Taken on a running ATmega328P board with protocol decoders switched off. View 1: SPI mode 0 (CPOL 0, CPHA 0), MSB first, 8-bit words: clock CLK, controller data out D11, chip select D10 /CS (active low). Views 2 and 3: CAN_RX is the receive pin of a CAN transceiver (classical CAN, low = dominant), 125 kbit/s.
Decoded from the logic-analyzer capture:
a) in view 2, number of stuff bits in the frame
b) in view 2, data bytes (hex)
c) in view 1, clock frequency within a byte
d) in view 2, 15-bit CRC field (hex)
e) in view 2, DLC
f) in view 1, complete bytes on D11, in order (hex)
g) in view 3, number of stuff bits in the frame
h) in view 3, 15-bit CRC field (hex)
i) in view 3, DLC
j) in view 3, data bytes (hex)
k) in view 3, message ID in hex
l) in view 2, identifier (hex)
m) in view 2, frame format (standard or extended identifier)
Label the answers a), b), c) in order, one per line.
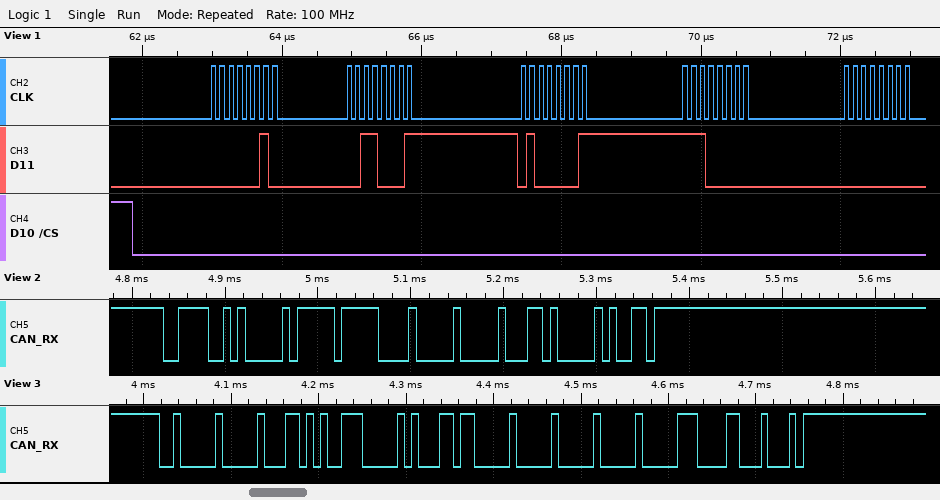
a) 6
b) FF 10 00
c) 8 MHz
d) 0x3409
e) 3
f) 02 31 41 E0 00
g) 8
h) 0x6188
i) 6
j) A7 02 36 00 00 00
k) 0x200
l) 0x3CA
m) standard
